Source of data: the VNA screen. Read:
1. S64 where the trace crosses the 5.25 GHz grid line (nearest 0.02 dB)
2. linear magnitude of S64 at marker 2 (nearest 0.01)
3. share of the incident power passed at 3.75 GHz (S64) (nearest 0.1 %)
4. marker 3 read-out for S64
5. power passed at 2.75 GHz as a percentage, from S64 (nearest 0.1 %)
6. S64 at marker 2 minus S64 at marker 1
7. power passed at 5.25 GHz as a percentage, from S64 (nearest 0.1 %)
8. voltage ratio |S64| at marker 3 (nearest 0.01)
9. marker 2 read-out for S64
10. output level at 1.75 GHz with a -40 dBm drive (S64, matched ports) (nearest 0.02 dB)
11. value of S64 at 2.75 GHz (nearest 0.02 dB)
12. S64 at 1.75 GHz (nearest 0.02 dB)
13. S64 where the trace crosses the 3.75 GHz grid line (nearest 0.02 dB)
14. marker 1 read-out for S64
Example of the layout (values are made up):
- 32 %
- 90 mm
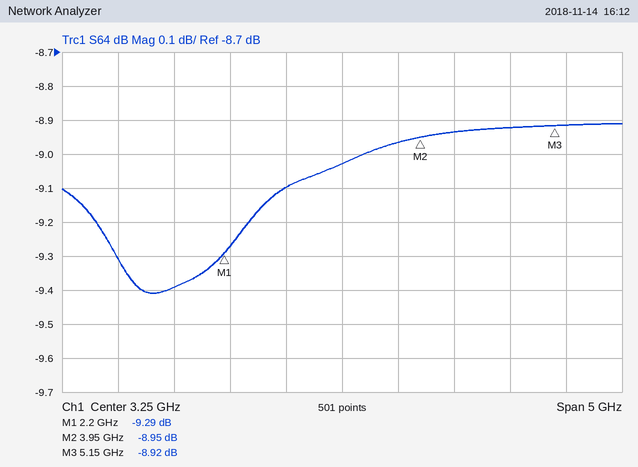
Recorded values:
- -8.92 dB
- 0.36
- 12.7 %
- -8.92 dB
- 12.3 %
- 0.34 dB
- 12.8 %
- 0.36
- -8.95 dB
- -49.40 dBm
- -9.10 dB
- -9.40 dB
- -8.96 dB
- -9.29 dB
